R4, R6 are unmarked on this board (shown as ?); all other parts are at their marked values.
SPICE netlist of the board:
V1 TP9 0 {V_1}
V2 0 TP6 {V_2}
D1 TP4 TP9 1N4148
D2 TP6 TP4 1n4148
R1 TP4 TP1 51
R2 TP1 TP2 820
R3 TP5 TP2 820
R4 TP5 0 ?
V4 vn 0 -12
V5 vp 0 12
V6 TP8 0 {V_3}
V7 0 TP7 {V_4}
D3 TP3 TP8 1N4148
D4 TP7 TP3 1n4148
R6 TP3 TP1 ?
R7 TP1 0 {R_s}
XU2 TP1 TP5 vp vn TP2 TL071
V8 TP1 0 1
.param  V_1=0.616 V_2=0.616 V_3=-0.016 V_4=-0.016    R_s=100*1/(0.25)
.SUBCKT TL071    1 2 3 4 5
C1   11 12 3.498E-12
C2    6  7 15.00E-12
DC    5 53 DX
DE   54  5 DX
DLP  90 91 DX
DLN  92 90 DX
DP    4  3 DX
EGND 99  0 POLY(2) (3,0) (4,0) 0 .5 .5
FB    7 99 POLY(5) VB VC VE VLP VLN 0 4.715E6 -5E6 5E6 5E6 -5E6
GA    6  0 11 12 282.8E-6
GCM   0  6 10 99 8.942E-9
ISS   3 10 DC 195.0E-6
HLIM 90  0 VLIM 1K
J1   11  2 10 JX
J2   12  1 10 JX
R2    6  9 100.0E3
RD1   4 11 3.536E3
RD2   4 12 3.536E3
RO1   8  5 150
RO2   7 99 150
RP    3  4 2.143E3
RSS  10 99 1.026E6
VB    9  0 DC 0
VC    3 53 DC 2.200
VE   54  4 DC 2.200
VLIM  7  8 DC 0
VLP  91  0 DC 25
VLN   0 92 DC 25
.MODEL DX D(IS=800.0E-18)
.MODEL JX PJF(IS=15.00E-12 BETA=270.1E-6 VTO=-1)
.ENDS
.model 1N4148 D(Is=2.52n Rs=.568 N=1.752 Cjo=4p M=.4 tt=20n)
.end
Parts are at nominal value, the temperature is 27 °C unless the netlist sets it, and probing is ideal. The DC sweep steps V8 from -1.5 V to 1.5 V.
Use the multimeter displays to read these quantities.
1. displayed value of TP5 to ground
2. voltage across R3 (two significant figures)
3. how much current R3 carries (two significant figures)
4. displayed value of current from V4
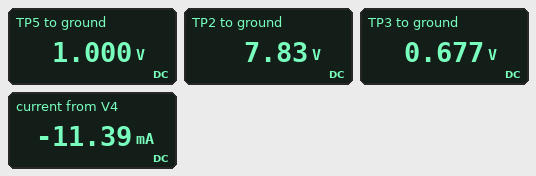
1.000 V
6.8 V
8.3 mA
-11.39 mA
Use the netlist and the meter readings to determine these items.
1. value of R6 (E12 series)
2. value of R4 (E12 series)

33 Ω
120 Ω
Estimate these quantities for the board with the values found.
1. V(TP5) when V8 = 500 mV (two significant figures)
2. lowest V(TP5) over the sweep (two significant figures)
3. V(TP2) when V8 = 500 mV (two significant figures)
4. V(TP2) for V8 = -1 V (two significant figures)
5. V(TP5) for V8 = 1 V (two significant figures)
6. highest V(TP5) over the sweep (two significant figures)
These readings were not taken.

500 mV
-1.3 V
3.9 V
-7.8 V
1.0 V
1.3 V
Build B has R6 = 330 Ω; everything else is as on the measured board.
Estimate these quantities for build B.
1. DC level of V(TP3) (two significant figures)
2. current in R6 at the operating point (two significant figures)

580 mV
1.3 mA
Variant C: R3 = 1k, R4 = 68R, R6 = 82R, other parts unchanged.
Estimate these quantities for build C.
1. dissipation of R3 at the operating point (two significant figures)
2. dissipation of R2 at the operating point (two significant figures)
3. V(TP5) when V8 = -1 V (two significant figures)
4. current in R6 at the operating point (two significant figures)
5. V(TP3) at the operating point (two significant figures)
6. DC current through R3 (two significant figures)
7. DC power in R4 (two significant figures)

96 mW
110 mW
-670 mV
4.4 mA
640 mV
9.8 mA
6.5 mW
